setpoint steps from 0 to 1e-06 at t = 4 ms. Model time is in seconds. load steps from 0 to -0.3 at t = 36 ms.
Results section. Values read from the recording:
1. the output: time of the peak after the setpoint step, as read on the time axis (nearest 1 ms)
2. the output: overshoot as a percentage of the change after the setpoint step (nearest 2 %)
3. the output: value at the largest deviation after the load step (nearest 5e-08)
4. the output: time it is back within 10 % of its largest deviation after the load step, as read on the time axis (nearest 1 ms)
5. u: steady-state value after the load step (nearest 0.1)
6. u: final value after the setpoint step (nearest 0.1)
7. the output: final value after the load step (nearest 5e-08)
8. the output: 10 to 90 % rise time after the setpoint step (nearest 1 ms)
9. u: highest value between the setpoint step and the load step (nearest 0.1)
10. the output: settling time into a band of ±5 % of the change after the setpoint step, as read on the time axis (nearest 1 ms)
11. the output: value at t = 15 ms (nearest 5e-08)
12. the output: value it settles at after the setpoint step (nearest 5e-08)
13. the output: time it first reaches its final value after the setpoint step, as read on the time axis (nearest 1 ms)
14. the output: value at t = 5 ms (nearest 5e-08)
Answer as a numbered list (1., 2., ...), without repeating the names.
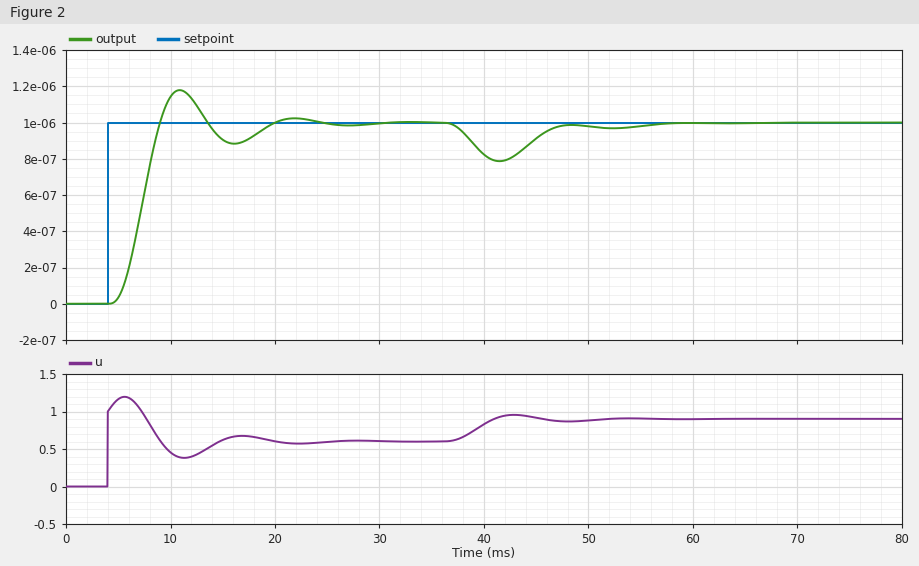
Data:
1. 11 ms
2. 18 %
3. 0.00000080
4. 55 ms
5. 0.9
6. 0.6
7. 0.00000100
8. 3 ms
9. 1.2
10. 19 ms
11. 0.00000090
12. 0.00000100
13. 9 ms
14. 0.00000005
